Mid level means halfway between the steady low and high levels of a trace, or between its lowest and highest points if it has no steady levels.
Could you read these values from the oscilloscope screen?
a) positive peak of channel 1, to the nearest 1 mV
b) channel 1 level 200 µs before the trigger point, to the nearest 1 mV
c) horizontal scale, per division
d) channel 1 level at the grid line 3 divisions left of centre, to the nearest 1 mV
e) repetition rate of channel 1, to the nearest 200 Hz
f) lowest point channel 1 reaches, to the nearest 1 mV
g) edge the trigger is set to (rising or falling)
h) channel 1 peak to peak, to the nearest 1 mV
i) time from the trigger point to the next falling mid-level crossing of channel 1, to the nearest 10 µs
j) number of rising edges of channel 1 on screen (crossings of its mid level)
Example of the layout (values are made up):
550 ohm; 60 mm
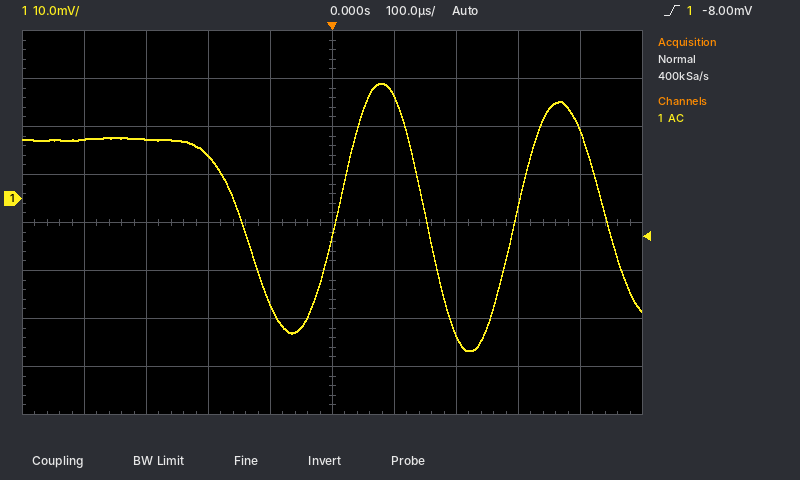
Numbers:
24 mV; 9 mV; 100 µs; 12 mV; 3.4 kHz; -32 mV; rising; 56 mV; 150 µs; 2
